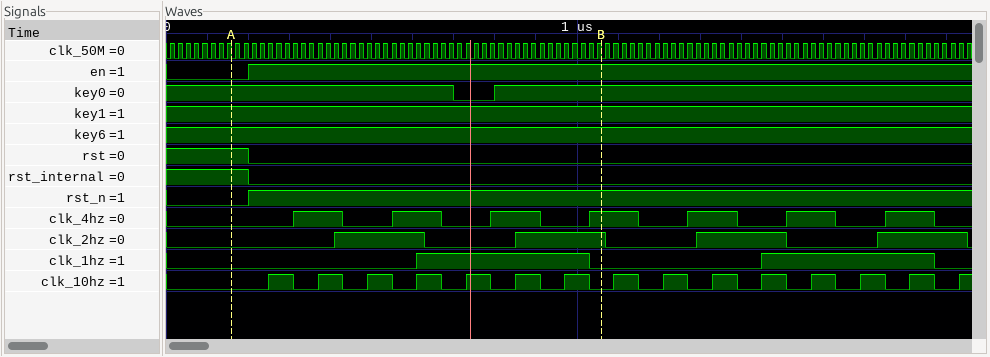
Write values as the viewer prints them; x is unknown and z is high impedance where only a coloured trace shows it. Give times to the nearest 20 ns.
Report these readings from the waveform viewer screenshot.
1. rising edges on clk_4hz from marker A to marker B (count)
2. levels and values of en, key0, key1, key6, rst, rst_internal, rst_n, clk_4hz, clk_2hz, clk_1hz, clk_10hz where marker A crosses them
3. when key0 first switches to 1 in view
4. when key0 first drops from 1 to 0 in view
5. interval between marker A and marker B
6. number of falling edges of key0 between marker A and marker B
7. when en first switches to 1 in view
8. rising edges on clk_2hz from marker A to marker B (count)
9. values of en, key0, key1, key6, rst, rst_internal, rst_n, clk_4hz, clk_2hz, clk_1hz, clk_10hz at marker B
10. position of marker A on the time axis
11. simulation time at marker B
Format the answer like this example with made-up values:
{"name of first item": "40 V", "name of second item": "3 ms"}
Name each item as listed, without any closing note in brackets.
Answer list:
{"rising edges on clk_4hz from marker A to marker B": "4", "levels and values of en, key0, key1, key6, rst, rst_internal, rst_n, clk_4hz, clk_2hz, clk_1hz, clk_10hz where marker A crosses them": "en=0, key0=1, key1=1, key6=1, rst=1, rst_internal=1, rst_n=0, clk_4hz=0, clk_2hz=0, clk_1hz=0, clk_10hz=0", "when key0 first switches to 1 in view": "800 ns", "when key0 first drops from 1 to 0 in view": "700 ns", "interval between marker A and marker B": "900 ns", "number of falling edges of key0 between marker A and marker B": "1", "when en first switches to 1 in view": "200 ns", "rising edges on clk_2hz from marker A to marker B": "2", "values of en, key0, key1, key6, rst, rst_internal, rst_n, clk_4hz, clk_2hz, clk_1hz, clk_10hz at marker B": "en=1, key0=1, key1=1, key6=1, rst=0, rst_internal=0, rst_n=1, clk_4hz=1, clk_2hz=1, clk_1hz=0, clk_10hz=0", "position of marker A on the time axis": "160 ns", "simulation time at marker B": "1060 ns"}
